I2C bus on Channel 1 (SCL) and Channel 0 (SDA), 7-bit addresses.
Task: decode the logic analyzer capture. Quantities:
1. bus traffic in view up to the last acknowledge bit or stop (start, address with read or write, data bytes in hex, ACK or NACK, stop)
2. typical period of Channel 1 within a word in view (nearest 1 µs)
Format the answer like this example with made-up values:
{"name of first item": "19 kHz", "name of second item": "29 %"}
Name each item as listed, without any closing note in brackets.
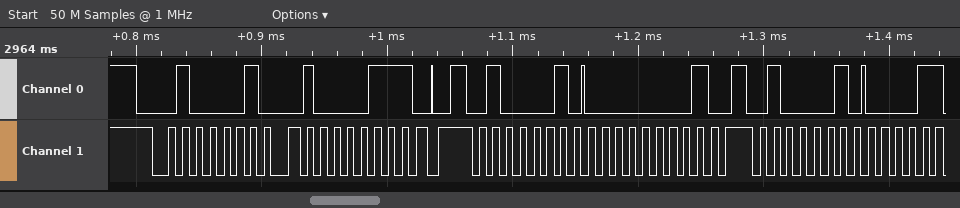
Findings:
{"bus traffic in view up to the last acknowledge bit or stop": "start, address 21 write ACK, 87 ACK, stop, start, address 21 write ACK, 01 ACK, stop, start, address 21 write ACK", "typical period of Channel 1 within a word in view": "11 µs"}
